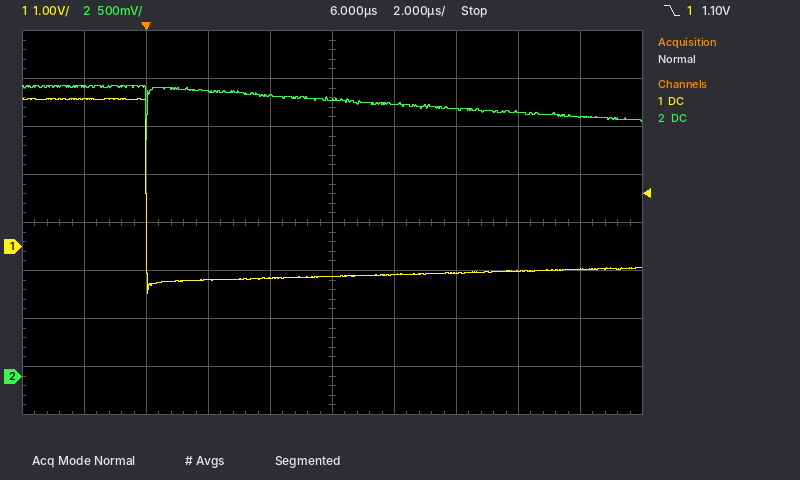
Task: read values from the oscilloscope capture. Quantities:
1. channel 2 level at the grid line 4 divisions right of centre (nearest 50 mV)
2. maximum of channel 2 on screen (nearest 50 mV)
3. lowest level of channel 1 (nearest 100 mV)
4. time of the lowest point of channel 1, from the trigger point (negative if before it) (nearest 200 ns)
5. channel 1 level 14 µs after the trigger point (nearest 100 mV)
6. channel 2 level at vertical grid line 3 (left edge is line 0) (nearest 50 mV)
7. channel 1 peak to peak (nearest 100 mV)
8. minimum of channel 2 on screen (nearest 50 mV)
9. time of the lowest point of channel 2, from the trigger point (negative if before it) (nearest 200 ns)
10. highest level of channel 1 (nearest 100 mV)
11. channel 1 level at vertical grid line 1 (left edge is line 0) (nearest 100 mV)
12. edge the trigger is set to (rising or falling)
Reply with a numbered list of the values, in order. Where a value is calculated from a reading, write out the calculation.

1. 2.70 V
2. 3.05 V
3. -1.0 V
4. 0.0 µs
5. -500 mV
6. 2.95 V
7. 3.1 V − (-1.0 V) = 4.1 V
8. 2.45 V
9. 0.0 µs
10. 3.1 V
11. 3.1 V
12. falling
